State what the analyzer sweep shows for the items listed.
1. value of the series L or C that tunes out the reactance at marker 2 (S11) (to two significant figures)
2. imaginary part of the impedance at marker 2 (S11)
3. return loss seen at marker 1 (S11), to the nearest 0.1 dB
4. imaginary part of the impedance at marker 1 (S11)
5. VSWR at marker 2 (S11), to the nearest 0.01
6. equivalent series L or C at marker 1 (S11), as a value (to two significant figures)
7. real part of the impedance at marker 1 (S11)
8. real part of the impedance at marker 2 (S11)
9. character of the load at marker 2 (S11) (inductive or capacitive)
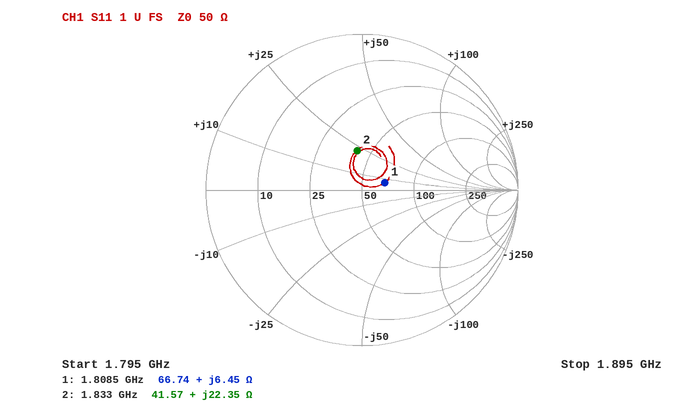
3.9 pF
+22.35 Ω
16.3 dB
+6.45 Ω
1.68
570 pH
66.74 Ω
41.57 Ω
inductive
